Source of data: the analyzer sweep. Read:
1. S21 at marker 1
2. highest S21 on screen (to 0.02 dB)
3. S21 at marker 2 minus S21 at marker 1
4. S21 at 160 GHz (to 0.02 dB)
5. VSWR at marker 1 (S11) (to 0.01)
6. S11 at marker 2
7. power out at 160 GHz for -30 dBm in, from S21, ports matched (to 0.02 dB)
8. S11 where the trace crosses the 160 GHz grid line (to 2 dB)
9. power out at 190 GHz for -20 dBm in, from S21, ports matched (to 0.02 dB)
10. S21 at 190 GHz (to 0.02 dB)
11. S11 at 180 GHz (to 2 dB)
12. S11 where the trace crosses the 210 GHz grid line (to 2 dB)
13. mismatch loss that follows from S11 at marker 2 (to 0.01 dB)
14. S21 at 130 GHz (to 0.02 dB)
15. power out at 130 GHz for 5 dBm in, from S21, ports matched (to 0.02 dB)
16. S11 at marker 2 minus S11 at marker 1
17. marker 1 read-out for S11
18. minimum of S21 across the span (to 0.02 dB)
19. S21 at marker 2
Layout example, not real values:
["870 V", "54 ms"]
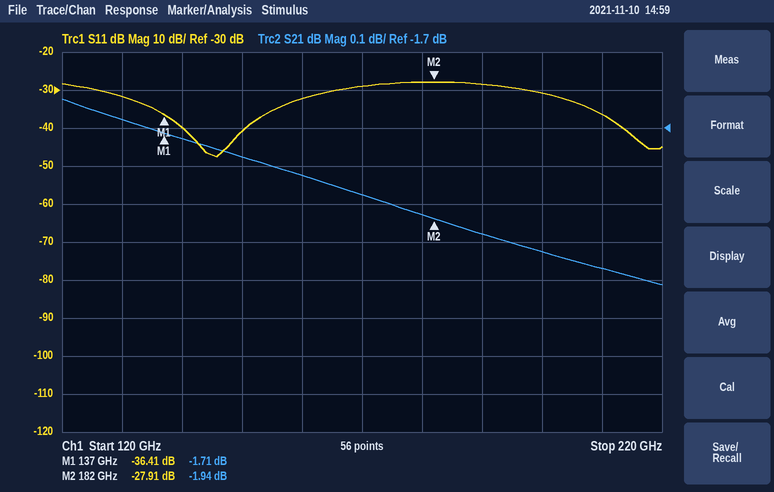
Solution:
["-1.71 dB", "-1.62 dB", "-0.23 dB", "-1.82 dB", "1.03", "-27.91 dB", "-31.82 dBm", "-32 dB", "-21.98 dBm", "-1.98 dB", "-28 dB", "-36 dB", "0.01 dB", "-1.68 dB", "3.32 dBm", "8.50 dB", "-36.41 dB", "-2.12 dB", "-1.94 dB"]
